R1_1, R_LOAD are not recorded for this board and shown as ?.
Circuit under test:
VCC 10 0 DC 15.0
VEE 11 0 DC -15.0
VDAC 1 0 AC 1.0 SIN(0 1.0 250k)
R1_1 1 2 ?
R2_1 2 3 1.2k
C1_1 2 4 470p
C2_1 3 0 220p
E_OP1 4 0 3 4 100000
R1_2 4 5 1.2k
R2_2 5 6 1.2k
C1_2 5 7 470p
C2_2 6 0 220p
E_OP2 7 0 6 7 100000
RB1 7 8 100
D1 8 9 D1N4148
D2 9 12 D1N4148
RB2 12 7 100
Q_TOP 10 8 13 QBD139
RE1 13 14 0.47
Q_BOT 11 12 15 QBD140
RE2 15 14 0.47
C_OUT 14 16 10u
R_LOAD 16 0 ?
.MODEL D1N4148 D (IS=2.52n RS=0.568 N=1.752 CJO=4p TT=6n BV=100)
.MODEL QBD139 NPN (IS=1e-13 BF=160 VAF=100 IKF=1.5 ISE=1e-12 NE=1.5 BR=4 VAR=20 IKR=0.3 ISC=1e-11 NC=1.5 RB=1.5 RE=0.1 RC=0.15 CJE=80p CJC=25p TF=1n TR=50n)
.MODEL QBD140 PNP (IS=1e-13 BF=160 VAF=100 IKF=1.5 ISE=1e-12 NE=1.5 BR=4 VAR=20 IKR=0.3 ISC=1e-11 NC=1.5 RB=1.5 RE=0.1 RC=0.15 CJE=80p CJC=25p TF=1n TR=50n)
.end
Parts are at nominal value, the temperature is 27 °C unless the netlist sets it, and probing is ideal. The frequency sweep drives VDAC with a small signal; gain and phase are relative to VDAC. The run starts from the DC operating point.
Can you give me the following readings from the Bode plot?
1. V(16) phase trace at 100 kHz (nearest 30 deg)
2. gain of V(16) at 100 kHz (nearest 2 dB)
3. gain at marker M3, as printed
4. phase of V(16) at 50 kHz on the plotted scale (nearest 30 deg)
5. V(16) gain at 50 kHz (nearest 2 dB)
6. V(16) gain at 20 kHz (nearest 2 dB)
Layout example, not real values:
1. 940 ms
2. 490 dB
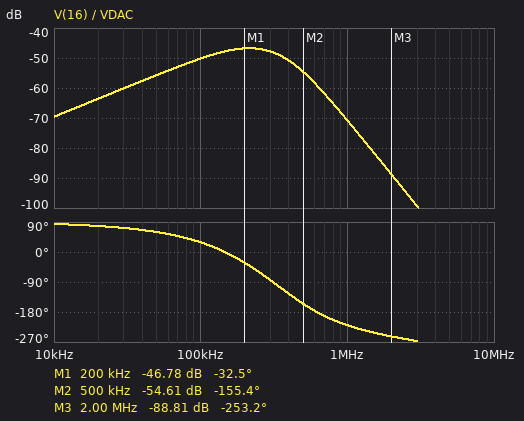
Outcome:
1. 30 deg
2. -50 dB
3. -88.81 dB
4. 60 deg
5. -56 dB
6. -64 dB
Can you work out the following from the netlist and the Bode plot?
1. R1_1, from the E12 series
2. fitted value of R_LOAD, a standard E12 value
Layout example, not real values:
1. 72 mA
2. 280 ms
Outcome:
1. 3.9 kΩ
2. 33 Ω
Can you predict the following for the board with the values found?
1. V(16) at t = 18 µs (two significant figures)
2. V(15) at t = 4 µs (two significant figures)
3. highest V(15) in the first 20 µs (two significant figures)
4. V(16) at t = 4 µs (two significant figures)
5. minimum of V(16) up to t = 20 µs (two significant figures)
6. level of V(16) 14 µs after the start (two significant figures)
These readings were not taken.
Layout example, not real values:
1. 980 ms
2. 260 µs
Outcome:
1. 4.0 mV
2. -4.0 mV
3. 24 mV
4. -4.0 mV
5. -5.1 mV
6. 4.0 mV
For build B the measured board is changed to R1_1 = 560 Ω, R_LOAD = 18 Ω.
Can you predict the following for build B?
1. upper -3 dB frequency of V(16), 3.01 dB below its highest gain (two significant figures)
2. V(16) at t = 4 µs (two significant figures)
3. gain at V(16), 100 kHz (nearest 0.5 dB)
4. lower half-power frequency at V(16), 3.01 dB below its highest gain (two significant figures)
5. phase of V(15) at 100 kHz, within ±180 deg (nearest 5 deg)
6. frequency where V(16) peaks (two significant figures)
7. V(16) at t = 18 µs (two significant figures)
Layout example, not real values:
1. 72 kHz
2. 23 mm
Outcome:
1. 580 kHz
2. -250 mV
3. -55.0 dB
4. 200 kHz
5. 55 deg
6. 360 kHz
7. 250 mV
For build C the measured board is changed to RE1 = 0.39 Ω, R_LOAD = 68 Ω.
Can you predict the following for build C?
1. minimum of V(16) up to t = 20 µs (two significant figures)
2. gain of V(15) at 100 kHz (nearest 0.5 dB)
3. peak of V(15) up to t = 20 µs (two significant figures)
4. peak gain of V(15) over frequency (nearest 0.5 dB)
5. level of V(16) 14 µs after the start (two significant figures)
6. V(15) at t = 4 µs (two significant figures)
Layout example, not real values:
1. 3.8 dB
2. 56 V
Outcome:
1. -9.4 mV
2. -44.0 dB
3. 34 mV
4. -40.5 dB
5. 8.3 mV
6. -8.3 mV
